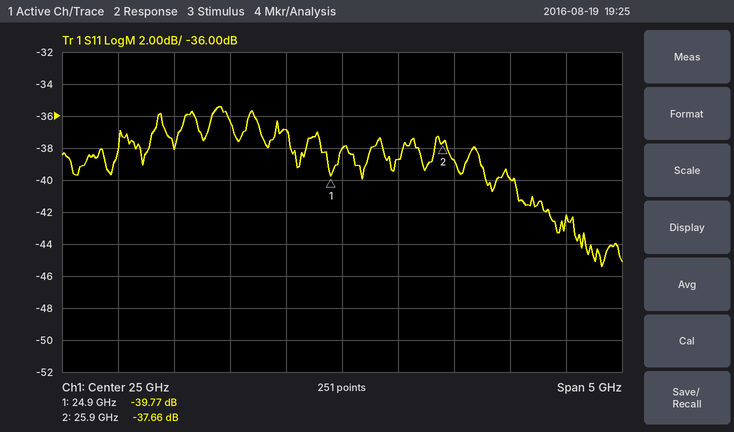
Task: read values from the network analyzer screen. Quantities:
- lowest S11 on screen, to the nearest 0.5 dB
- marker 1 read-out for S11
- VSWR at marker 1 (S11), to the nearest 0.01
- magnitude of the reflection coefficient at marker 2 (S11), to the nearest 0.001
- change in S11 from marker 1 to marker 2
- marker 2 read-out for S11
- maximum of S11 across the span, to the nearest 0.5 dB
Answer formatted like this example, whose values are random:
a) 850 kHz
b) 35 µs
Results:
a) -45.5 dB
b) -39.77 dB
c) 1.02
d) 0.013
e) 2.11 dB
f) -37.66 dB
g) -35.5 dB
